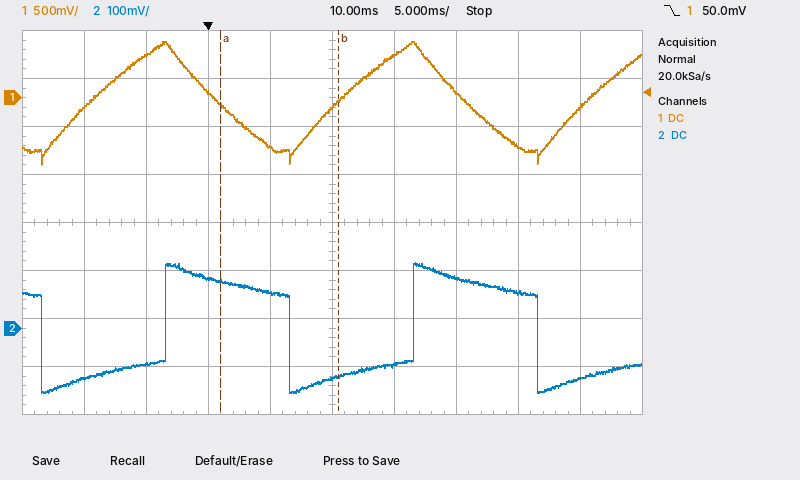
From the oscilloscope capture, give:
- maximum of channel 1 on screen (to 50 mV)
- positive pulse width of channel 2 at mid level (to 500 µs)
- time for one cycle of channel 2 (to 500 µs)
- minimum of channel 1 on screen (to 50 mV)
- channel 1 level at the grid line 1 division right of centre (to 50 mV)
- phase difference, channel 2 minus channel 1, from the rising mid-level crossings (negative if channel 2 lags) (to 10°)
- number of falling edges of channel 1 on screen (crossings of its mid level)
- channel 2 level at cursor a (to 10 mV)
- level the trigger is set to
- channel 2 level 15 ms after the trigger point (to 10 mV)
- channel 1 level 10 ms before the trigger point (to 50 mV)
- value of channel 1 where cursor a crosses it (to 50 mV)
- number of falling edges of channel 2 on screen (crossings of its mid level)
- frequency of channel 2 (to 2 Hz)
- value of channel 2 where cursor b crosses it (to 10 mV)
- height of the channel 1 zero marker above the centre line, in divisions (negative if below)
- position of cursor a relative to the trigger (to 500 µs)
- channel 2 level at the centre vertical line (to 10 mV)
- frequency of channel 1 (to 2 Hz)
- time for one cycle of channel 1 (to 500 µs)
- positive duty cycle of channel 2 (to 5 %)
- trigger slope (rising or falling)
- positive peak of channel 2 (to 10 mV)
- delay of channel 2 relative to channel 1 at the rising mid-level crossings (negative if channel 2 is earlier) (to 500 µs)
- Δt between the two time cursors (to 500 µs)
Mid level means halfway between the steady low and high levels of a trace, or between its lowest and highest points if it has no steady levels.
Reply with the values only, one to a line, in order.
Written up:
600 mV
10.0 ms
20.0 ms
-700 mV
450 mV
-110°
2
100 mV
50.0 mV
-80 mV
-100 mV
-50 mV
3
50 Hz
-100 mV
+2.6 div
+1.0 ms
-100 mV
50 Hz
20.0 ms
50 %
falling
140 mV
+6.0 ms
9.5 ms
